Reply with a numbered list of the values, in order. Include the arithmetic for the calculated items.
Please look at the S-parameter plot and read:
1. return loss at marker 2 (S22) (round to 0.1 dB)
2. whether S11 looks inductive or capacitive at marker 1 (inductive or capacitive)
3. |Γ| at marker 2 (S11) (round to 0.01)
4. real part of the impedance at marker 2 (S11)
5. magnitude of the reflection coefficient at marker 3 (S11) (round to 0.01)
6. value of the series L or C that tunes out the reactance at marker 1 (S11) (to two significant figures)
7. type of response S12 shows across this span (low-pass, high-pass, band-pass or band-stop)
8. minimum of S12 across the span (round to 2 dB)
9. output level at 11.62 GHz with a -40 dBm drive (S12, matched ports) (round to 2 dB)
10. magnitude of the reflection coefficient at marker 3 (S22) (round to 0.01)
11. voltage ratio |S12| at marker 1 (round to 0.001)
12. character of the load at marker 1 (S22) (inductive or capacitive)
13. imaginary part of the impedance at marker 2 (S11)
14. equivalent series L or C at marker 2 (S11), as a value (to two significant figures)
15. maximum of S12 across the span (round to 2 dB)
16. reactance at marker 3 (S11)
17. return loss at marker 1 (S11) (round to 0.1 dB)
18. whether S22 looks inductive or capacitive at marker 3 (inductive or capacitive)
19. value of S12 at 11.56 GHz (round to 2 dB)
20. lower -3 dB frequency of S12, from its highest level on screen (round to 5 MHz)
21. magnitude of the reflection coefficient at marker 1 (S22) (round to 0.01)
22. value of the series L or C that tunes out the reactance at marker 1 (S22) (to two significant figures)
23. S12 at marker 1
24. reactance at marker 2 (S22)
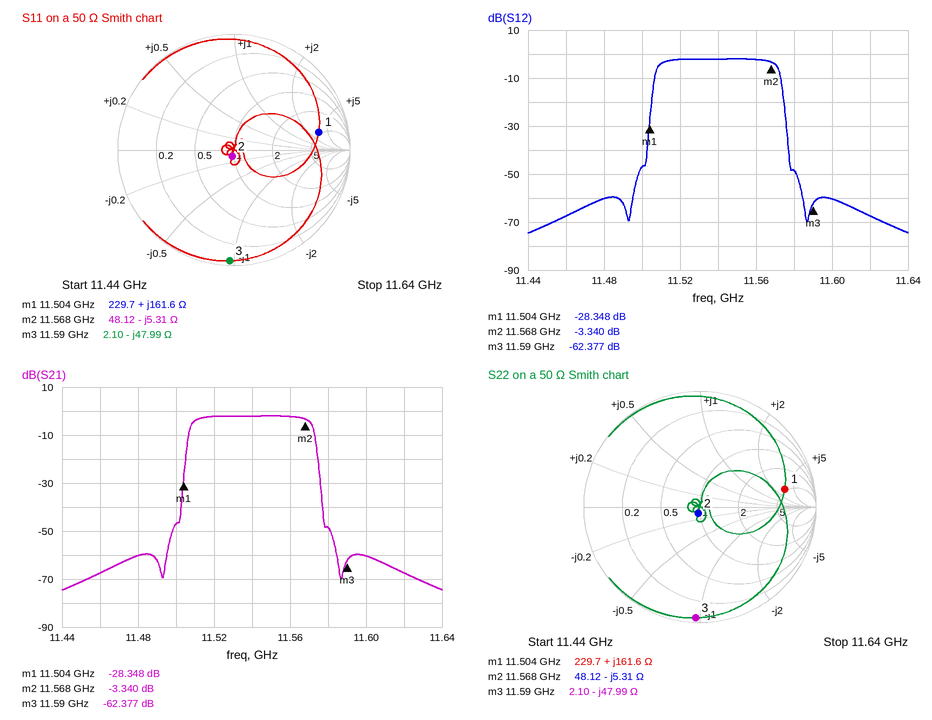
1. 24.8 dB
2. inductive
3. 0.06
4. 48.12 Ω
5. 0.96
6. C = 1/(2π × 11.504 GHz × 161.6 Ω) ≈ 86 fF
7. band-pass
8. -74 dB
9. -40 dBm + (-68 dB) = -108 dBm
10. 0.96
11. 10^(-28.348/20) ≈ 0.038
12. inductive
13. -5.31 Ω
14. C = 1/(2π × 11.568 GHz × 5.31 Ω) ≈ 2.6 pF
15. -2 dB
16. -47.99 Ω
17. 2.5 dB
18. capacitive
19. -2 dB
20. 11.510 GHz
21. 0.75
22. C = 1/(2π × 11.504 GHz × 161.6 Ω) ≈ 86 fF
23. -28.348 dB
24. -5.31 Ω
